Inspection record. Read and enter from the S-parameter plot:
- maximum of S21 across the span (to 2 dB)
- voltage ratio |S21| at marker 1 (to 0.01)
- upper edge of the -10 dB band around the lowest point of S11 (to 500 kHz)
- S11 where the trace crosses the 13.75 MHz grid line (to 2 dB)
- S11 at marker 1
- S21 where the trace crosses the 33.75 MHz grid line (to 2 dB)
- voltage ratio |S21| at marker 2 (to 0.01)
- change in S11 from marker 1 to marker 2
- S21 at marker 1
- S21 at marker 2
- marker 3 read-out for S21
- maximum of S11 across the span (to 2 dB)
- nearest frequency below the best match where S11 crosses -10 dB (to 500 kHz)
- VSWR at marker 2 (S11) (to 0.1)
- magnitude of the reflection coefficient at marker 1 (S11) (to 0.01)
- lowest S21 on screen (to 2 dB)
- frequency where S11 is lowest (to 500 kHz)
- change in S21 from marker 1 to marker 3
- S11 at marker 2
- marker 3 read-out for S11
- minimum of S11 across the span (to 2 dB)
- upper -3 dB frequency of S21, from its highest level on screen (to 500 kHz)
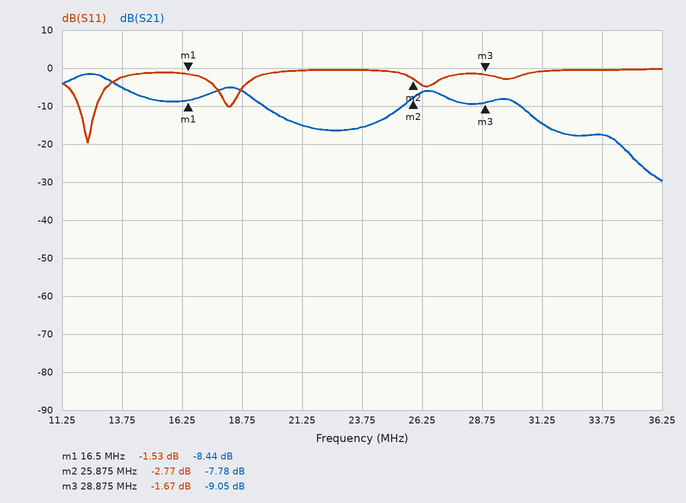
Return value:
-2 dB
0.38
12.5 MHz
-2 dB
-1.53 dB
-18 dB
0.41
-1.24 dB
-8.44 dB
-7.78 dB
-9.05 dB
0 dB
12.0 MHz
6.3
0.84
-30 dB
12.5 MHz
-0.61 dB
-2.77 dB
-1.67 dB
-20 dB
13.5 MHz
